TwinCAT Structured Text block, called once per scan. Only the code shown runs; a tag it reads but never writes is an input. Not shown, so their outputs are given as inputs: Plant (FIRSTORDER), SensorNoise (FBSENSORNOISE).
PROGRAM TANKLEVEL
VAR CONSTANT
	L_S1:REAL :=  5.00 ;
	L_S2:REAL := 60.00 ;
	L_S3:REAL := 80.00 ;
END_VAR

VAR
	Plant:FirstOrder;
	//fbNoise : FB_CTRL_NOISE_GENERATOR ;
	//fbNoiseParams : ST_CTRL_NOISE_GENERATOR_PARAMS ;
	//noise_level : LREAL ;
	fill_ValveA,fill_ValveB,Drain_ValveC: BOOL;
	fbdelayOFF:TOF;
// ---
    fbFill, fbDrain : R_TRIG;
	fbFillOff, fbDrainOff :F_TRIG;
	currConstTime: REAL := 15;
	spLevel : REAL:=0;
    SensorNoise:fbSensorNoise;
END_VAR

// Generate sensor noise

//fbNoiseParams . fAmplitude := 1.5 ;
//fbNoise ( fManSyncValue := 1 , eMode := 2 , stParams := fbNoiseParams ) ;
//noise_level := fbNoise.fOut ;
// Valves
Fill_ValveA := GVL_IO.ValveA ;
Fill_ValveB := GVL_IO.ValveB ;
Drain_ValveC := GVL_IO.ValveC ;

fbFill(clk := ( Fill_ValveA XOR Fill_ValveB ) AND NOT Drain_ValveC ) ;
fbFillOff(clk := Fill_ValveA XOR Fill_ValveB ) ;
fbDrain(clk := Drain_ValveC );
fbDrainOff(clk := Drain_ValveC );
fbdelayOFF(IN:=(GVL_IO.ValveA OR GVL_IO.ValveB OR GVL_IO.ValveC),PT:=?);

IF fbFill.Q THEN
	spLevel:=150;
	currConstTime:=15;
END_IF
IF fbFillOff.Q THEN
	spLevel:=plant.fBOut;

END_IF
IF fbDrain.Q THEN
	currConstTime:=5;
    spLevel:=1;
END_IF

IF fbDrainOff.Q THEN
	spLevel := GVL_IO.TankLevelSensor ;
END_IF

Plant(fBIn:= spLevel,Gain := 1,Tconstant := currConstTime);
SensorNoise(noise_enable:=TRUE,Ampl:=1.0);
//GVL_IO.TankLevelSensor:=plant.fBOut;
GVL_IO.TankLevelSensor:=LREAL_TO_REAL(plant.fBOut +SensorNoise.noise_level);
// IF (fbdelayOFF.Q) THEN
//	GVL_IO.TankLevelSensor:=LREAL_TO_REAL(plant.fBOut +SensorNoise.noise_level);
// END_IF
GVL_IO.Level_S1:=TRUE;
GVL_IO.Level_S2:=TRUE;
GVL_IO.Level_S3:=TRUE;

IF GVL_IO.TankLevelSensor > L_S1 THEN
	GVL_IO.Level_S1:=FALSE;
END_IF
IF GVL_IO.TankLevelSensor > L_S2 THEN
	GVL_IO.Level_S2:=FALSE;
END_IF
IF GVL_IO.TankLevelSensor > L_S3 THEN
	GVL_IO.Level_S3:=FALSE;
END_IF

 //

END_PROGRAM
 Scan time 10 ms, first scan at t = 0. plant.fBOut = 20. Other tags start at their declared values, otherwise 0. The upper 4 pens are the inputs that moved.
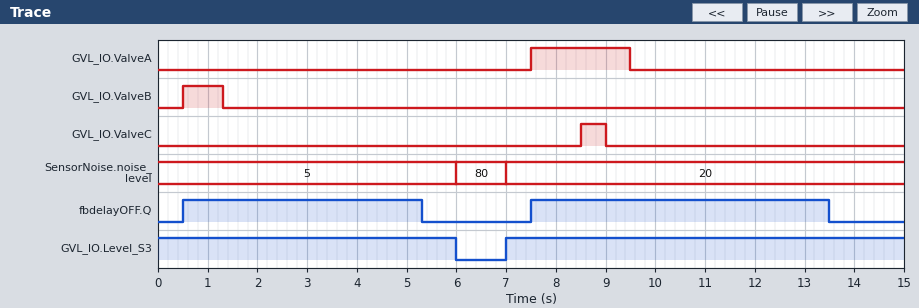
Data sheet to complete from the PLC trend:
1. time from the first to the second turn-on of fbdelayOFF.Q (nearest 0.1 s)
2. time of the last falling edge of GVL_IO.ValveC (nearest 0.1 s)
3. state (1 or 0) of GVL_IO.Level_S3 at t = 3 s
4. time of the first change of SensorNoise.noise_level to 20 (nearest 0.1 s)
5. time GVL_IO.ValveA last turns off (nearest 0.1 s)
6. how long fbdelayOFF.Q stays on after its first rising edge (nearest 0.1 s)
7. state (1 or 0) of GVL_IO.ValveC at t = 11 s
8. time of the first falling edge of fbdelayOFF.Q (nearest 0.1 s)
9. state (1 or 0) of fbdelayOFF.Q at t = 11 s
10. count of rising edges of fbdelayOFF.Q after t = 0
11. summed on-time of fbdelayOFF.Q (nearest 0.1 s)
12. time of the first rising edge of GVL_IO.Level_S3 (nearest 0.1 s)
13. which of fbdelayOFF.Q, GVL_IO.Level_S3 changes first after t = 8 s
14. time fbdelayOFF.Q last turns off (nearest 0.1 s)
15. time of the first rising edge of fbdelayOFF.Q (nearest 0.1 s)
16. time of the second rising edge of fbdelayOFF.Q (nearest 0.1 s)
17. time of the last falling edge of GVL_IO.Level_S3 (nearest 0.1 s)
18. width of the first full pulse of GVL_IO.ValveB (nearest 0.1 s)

7.0 s
9.0 s
1
7.0 s
9.5 s
4.8 s
0
5.3 s
1
2
10.8 s
7.0 s
fbdelayOFF.Q
13.5 s
0.5 s
7.5 s
6.0 s
0.8 s
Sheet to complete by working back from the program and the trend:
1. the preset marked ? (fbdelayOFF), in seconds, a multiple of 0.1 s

4.0 s
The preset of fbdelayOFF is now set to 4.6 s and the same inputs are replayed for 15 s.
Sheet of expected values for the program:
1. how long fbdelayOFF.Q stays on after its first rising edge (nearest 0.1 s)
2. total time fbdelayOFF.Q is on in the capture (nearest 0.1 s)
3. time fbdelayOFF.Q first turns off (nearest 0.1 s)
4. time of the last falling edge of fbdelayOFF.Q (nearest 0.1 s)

5.4 s
12.0 s
5.9 s
14.1 s
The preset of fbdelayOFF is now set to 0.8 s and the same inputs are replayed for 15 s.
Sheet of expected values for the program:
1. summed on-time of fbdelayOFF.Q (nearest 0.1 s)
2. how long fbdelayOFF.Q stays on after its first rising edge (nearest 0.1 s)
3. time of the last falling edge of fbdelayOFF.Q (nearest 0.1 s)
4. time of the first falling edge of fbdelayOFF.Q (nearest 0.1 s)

4.4 s
1.6 s
10.3 s
2.1 s
